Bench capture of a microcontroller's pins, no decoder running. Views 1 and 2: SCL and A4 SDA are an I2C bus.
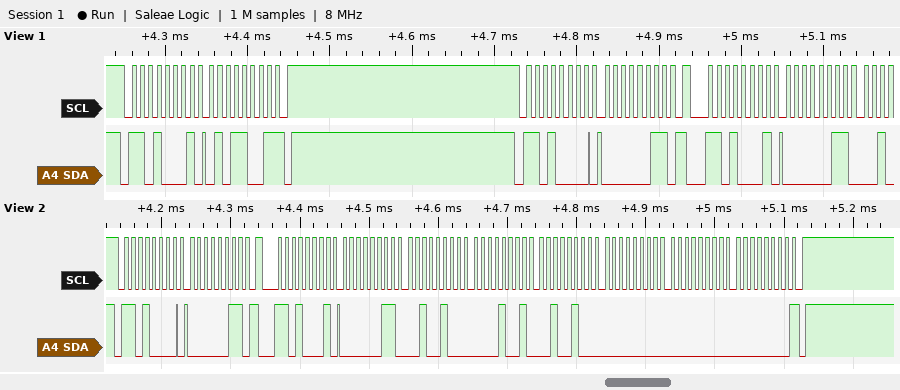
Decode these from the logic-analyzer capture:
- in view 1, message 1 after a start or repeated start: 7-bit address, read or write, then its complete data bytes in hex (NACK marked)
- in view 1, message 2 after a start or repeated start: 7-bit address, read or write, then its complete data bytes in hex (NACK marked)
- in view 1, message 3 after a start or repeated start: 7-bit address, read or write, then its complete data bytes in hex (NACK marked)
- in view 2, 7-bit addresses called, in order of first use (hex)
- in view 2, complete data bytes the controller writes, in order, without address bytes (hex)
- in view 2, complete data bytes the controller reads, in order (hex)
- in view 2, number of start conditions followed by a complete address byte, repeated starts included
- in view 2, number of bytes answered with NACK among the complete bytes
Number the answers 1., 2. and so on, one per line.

1. 0x68 read: 59 NACK
2. 0x68 write: 03
3. 0x68 read: 03
4. 0x68
5. 03
6. 03 24 09 24 00 00 00
7. 2
8. 1
